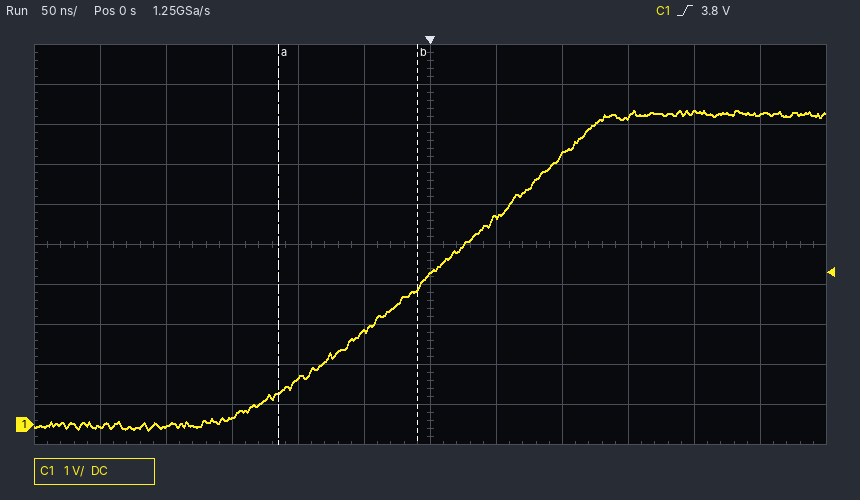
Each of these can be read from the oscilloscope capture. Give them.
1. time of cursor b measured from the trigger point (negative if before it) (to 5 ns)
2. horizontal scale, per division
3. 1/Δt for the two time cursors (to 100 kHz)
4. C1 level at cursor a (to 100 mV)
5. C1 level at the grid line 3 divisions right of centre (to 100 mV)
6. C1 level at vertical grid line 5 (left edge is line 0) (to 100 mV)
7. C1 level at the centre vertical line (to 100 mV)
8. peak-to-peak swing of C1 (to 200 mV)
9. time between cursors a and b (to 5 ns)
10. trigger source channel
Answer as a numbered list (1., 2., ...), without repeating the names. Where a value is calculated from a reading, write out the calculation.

1. -10 ns
2. 50 ns
3. 1 / 105 ns ≈ 9.5 MHz
4. 800 mV
5. 7.7 V
6. 2.3 V
7. 3.8 V
8. 8.0 V
9. 105 ns
10. C1
